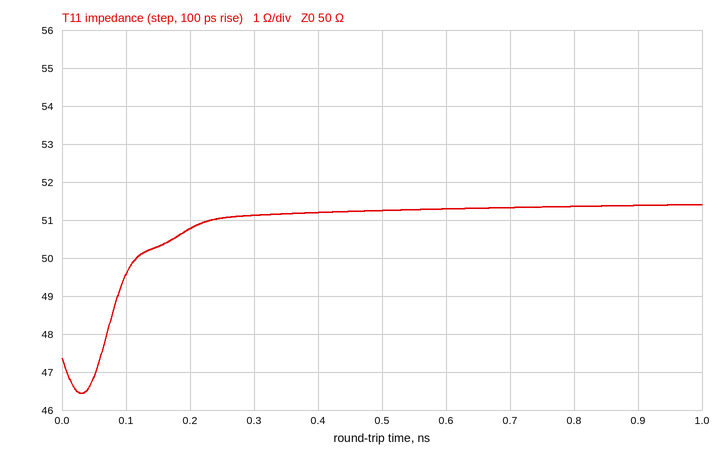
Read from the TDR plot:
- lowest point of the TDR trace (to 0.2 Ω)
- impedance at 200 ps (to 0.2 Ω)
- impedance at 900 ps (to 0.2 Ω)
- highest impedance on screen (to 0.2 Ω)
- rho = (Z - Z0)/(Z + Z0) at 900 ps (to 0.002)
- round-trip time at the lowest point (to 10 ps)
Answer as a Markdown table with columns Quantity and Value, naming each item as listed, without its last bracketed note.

| Quantity | Value |
|---|---|
| lowest point of the TDR trace | 46.4 Ω |
| impedance at 200 ps | 50.8 Ω |
| impedance at 900 ps | 51.4 Ω |
| highest impedance on screen | 51.4 Ω |
| rho = (Z - Z0)/(Z + Z0) at 900 ps | +0.014 |
| round-trip time at the lowest point | 30 ps |
